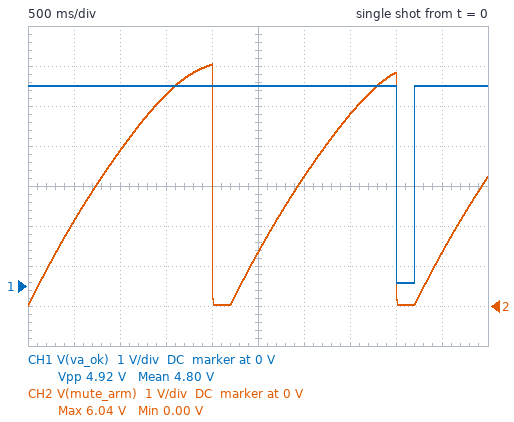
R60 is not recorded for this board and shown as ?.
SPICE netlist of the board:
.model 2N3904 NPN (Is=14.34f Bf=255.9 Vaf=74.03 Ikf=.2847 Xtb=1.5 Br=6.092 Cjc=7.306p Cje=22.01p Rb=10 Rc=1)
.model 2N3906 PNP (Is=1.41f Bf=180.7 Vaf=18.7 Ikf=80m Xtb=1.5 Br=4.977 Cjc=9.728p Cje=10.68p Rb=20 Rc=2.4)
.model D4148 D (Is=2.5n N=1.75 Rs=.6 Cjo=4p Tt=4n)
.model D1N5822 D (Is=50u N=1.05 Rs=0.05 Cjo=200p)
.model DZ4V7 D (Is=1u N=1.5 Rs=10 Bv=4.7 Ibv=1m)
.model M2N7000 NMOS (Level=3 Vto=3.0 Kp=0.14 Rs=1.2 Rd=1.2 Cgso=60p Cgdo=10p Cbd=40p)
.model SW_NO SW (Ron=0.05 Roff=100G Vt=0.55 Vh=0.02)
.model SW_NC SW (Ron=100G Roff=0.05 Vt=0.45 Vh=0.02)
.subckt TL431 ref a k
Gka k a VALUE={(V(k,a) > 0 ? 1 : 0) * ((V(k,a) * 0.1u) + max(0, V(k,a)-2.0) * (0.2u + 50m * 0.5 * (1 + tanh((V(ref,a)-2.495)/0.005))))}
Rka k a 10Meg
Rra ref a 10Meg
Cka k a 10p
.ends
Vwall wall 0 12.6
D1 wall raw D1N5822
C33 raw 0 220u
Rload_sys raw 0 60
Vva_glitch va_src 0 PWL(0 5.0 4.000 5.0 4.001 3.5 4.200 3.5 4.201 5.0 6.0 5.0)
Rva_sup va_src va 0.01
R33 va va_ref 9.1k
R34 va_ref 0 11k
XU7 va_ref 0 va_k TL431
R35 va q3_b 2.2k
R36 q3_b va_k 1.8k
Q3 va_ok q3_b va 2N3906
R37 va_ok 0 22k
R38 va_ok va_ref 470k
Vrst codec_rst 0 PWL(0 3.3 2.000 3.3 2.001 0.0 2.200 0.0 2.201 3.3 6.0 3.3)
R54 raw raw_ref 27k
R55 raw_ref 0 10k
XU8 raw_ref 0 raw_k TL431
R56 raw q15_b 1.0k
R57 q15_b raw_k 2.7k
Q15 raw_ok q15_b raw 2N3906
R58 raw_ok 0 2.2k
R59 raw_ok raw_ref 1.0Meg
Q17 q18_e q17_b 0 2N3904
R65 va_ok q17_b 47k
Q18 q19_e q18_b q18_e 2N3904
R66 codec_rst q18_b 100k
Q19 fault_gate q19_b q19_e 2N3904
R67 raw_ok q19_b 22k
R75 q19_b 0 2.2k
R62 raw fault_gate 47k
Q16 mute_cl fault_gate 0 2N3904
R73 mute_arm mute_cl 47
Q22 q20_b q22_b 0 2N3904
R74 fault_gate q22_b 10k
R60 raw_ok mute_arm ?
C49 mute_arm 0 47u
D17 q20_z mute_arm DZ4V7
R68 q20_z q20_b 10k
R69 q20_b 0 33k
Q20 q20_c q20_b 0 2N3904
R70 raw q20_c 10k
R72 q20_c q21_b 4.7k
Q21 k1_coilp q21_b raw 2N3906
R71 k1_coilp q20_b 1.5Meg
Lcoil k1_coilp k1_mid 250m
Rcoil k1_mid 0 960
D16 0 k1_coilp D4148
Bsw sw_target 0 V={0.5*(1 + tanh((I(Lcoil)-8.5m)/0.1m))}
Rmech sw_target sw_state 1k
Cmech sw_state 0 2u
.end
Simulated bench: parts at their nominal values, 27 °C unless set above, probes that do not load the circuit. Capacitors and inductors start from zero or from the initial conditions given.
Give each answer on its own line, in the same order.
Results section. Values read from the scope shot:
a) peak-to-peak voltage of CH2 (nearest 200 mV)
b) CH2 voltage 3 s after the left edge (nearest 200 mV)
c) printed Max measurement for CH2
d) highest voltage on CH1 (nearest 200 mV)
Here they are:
6.0 V
3.2 V
6.04 V
5.0 V
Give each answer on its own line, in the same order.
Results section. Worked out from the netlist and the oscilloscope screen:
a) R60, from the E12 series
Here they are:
56 kΩ
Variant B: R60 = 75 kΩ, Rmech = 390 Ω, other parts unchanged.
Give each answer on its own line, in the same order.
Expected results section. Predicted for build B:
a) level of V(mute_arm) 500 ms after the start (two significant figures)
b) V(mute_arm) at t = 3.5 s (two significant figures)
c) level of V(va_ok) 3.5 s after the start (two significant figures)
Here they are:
1.6 V
3.8 V
5.0 V
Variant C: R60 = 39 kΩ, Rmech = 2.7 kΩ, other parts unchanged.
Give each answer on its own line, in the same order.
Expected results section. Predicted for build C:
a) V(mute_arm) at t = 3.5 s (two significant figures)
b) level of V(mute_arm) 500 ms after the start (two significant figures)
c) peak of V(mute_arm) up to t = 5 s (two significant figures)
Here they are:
6.0 V
2.9 V
6.6 V
